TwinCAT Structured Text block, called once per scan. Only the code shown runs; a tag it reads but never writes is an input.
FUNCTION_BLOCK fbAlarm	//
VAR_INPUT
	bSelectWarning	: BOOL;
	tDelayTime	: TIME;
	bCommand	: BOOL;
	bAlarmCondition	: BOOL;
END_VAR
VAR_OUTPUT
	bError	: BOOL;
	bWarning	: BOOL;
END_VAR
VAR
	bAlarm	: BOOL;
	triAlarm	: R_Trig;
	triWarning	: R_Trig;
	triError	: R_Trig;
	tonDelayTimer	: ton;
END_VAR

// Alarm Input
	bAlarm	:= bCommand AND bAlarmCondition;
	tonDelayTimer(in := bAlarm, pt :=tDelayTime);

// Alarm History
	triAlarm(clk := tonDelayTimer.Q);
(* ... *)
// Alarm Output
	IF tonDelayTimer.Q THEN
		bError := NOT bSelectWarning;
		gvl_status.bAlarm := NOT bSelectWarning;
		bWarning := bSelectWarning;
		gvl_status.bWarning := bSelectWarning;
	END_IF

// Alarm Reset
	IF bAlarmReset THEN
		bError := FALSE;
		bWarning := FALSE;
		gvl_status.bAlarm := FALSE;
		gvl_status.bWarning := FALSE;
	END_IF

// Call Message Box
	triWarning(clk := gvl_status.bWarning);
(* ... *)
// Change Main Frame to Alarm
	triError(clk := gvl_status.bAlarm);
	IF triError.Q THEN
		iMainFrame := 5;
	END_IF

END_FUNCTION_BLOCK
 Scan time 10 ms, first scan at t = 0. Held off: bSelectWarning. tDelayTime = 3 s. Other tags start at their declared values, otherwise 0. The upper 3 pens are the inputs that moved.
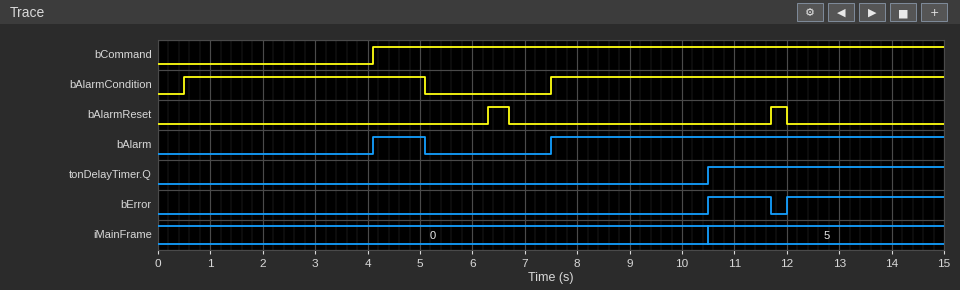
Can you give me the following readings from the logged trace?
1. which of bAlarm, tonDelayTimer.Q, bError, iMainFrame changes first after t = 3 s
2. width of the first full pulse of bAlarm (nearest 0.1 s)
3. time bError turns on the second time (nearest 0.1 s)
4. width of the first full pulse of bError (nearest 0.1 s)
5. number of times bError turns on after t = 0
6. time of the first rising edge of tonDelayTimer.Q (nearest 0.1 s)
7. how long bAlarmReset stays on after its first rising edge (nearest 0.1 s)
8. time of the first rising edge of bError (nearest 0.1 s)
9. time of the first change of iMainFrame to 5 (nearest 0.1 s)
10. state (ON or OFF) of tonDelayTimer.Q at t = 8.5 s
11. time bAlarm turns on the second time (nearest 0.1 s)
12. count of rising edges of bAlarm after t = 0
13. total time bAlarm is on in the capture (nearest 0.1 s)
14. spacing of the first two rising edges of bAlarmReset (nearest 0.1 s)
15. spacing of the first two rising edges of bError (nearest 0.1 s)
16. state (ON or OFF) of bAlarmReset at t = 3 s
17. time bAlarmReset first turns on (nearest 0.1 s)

bAlarm
1.0 s
12.0 s
1.2 s
2
10.5 s
0.4 s
10.5 s
10.5 s
OFF
7.5 s
2
8.5 s
5.4 s
1.5 s
OFF
6.3 s
